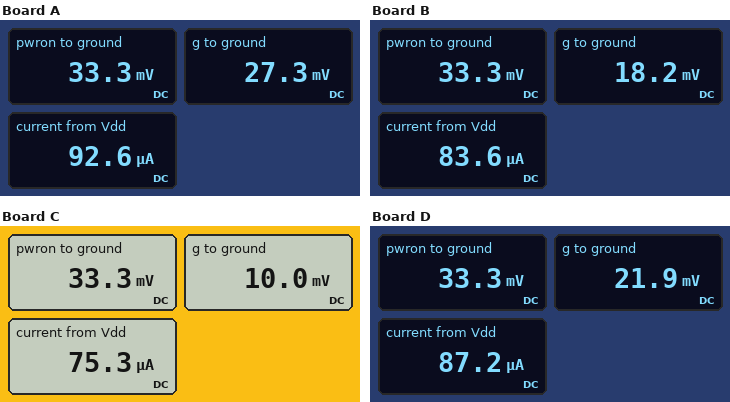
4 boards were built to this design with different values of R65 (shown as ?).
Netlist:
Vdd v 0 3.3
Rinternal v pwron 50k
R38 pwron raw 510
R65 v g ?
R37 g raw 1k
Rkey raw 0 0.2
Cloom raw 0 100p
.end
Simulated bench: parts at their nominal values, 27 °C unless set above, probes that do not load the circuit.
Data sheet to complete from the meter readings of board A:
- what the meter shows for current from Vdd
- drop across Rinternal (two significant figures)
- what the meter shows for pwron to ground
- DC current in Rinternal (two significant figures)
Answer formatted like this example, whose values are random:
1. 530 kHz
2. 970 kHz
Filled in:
1. 92.6 µA
2. 3.3 V
3. 33.3 mV
4. 65 µA
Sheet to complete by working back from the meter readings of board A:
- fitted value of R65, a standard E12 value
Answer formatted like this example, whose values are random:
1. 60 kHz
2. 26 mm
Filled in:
1. 120 kΩ
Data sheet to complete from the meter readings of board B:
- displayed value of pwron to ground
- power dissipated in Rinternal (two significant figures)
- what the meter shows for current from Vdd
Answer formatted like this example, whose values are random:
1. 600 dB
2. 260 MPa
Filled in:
1. 33.3 mV
2. 210 µW
3. 83.6 µA
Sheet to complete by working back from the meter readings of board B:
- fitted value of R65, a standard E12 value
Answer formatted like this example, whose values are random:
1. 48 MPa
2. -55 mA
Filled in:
1. 180 kΩ
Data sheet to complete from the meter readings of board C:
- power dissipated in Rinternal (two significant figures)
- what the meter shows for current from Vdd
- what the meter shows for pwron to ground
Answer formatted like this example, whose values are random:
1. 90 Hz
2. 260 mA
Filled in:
1. 210 µW
2. 75.3 µA
3. 33.3 mV
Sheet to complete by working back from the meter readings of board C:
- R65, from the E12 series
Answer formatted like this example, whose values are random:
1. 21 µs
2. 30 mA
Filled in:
1. 330 kΩ
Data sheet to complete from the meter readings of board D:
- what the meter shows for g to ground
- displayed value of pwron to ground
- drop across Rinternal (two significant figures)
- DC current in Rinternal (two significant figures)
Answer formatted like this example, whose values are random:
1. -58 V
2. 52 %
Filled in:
1. 21.9 mV
2. 33.3 mV
3. 3.3 V
4. 65 µA
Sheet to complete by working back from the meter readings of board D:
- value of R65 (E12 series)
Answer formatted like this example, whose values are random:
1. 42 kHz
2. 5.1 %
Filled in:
1. 150 kΩ
